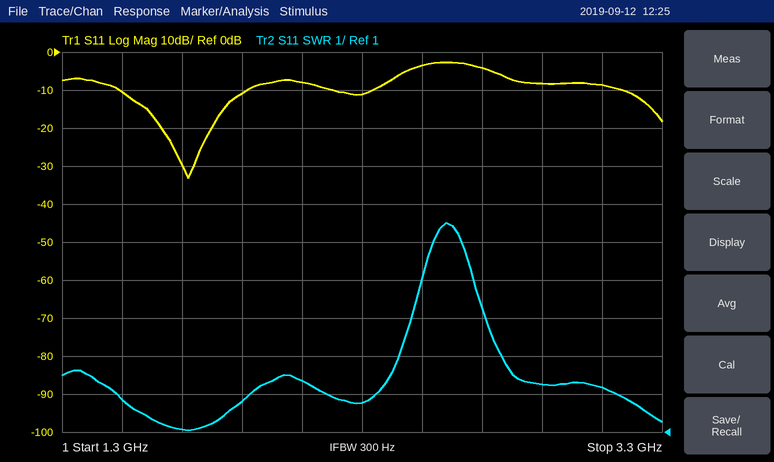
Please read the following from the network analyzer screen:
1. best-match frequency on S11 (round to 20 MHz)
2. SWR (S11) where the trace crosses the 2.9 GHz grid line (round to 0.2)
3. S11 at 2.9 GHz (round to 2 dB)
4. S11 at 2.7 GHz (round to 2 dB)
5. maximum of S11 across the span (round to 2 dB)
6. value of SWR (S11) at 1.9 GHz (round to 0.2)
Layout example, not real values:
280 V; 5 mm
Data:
1.72 GHz; 2.2; -8 dB; -4 dB; -2 dB; 1.8
